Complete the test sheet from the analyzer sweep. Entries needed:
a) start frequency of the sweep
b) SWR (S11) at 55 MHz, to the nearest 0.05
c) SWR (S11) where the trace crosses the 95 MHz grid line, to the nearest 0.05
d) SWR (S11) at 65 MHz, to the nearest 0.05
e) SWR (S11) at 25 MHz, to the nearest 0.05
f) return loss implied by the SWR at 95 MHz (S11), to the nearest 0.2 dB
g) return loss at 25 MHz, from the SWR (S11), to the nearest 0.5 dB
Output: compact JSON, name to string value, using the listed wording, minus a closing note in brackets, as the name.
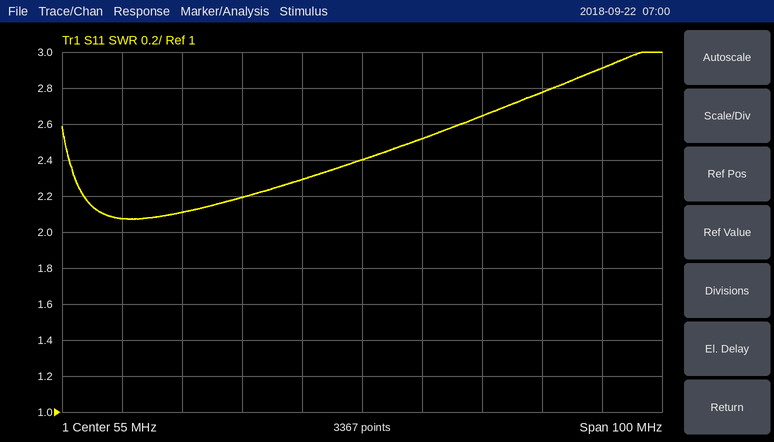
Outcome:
{"start frequency of the sweep": "5 MHz", "SWR (S11) at 55 MHz, to the nearest 0.05": "2.40", "SWR (S11) where the trace crosses the 95 MHz grid line, to the nearest 0.05": "2.90", "SWR (S11) at 65 MHz, to the nearest 0.05": "2.50", "SWR (S11) at 25 MHz, to the nearest 0.05": "2.10", "return loss implied by the SWR at 95 MHz (S11), to the nearest 0.2 dB": "6.2 dB", "return loss at 25 MHz, from the SWR (S11), to the nearest 0.5 dB": "9.0 dB"}
